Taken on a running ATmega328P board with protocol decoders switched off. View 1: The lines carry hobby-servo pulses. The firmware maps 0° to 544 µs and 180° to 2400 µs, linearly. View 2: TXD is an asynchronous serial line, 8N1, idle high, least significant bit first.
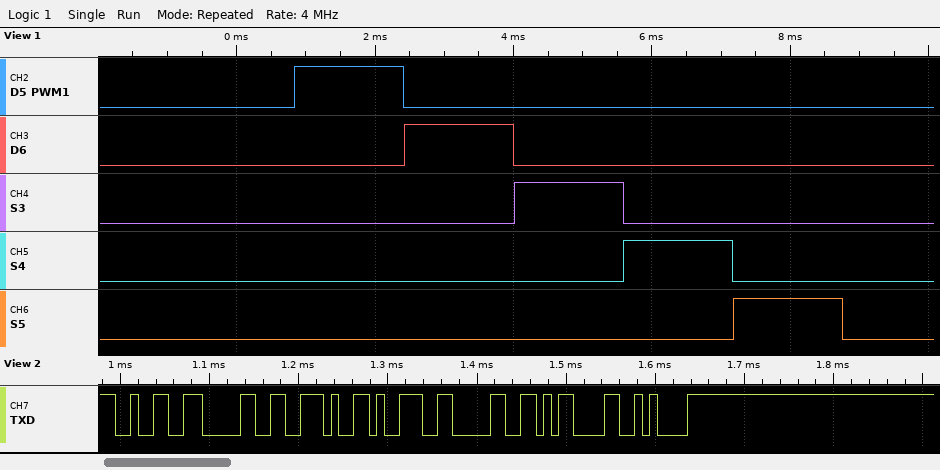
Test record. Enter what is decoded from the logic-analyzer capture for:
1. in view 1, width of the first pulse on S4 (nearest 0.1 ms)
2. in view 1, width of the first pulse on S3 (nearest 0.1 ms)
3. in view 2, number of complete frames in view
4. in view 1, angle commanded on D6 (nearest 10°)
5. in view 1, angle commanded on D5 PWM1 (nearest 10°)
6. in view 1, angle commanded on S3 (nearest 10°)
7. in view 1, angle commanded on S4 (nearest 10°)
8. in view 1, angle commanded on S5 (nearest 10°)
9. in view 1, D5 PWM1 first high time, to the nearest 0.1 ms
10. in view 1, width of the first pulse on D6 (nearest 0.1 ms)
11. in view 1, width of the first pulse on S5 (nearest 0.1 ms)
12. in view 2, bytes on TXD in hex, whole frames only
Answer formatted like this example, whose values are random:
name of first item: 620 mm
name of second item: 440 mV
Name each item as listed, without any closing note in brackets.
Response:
in view 1, width of the first pulse on S4: 1.6 ms
in view 1, width of the first pulse on S3: 1.6 ms
in view 2, number of complete frames in view: 7
in view 1, angle commanded on D6: 100°
in view 1, angle commanded on D5 PWM1: 100°
in view 1, angle commanded on S3: 100°
in view 1, angle commanded on S4: 100°
in view 1, angle commanded on S5: 100°
in view 1, D5 PWM1 first high time, to the nearest 0.1 ms: 1.6 ms
in view 1, width of the first pulse on D6: 1.6 ms
in view 1, width of the first pulse on S5: 1.6 ms
in view 2, bytes on TXD in hex, whole frames only: 32 30 2E 39 30 0D 0A
